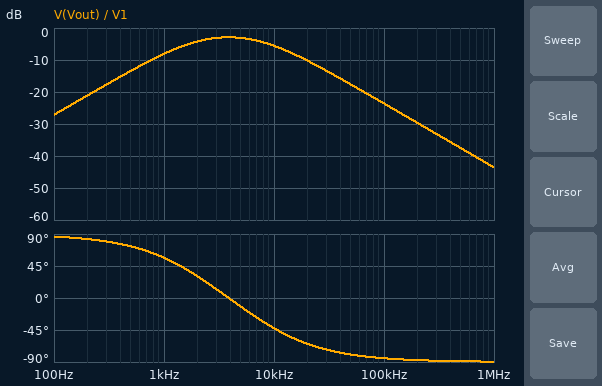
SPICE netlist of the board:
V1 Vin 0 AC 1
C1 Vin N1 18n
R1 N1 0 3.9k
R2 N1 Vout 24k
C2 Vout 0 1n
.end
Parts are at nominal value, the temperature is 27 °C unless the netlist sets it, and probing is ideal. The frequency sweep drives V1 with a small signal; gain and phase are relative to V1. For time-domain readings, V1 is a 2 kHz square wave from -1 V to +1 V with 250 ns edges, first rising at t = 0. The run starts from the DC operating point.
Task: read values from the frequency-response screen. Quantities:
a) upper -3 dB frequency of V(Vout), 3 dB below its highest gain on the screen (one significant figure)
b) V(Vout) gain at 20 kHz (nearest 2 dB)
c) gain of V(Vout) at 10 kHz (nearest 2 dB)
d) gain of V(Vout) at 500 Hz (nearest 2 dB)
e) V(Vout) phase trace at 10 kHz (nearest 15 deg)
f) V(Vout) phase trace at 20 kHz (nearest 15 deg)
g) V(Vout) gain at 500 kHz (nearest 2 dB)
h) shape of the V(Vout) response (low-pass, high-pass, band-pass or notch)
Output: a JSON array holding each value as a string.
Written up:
["10 kHz", "-10 dB", "-6 dB", "-14 dB", "-45 deg", "-60 deg", "-38 dB", "band-pass"]
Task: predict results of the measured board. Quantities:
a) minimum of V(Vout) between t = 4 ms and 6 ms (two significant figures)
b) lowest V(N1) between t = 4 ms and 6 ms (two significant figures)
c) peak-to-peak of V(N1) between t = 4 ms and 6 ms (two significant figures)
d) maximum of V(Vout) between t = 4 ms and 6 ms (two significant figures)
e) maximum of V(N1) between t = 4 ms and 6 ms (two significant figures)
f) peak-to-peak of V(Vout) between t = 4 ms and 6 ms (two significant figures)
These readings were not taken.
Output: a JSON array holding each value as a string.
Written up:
["-1.1 V", "-1.9 V", "3.9 V", "1.1 V", "1.9 V", "2.1 V"]
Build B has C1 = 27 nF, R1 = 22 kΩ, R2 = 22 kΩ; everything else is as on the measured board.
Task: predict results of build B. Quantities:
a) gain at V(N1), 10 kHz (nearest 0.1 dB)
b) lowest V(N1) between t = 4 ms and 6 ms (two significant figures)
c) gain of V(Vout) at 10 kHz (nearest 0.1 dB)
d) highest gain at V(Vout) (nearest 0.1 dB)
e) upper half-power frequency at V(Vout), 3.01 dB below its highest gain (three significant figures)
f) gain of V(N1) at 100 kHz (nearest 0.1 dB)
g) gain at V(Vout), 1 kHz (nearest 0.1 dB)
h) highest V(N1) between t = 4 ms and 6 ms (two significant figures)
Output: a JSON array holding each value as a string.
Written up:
["-0.1 dB", "-1.2 V", "-4.8 dB", "-0.6 dB", "8.01 kHz", "0 dB", "-0.7 dB", "1.2 V"]
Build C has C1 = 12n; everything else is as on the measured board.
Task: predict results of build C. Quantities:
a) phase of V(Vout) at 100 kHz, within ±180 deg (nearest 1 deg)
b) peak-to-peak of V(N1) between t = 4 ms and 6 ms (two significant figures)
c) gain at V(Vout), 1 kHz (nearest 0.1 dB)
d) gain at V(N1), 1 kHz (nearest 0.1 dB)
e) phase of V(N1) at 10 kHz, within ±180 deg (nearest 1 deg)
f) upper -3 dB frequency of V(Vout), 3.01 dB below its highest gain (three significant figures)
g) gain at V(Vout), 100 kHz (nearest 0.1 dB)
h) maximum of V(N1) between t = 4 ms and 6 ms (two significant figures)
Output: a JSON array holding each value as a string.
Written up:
["-84 deg", "4.0 V", "-11.2 dB", "-11.1 dB", "20 deg", "12.4 kHz", "-23.6 dB", "2.0 V"]
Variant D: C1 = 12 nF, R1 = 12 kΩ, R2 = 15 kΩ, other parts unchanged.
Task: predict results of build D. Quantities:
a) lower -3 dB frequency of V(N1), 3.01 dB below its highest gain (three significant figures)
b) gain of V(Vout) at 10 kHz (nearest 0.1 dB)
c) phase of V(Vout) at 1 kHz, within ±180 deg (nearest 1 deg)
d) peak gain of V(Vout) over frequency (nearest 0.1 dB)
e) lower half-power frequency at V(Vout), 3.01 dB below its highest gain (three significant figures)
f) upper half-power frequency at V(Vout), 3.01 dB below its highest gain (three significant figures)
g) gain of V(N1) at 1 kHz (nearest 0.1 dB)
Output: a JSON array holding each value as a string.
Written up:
["1.23 kHz", "-3.2 dB", "40 deg", "-1.5 dB", "871 Hz", "13.5 kHz", "-3.8 dB"]
